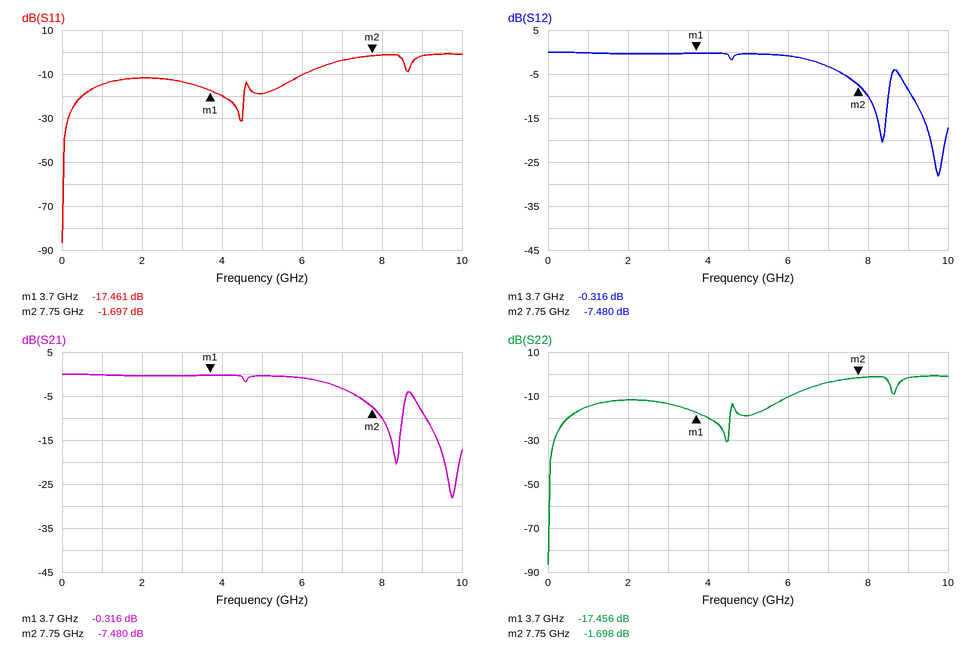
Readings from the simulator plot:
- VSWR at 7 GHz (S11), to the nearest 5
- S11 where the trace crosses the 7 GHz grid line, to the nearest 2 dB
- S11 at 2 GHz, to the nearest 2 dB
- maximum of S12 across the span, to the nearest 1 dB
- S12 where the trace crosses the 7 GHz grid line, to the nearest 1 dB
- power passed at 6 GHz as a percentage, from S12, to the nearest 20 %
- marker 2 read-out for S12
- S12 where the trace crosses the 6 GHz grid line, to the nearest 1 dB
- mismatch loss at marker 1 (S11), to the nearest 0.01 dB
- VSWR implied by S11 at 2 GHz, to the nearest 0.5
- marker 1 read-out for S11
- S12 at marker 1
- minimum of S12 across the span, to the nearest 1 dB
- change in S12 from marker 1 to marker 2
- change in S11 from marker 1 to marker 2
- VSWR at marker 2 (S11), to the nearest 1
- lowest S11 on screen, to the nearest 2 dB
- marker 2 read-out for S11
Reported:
5
-4 dB
-12 dB
0 dB
-3 dB
80 %
-7.480 dB
-1 dB
0.08 dB
1.5
-17.461 dB
-0.316 dB
-28 dB
-7.164 dB
15.764 dB
10
-86 dB
-1.697 dB
